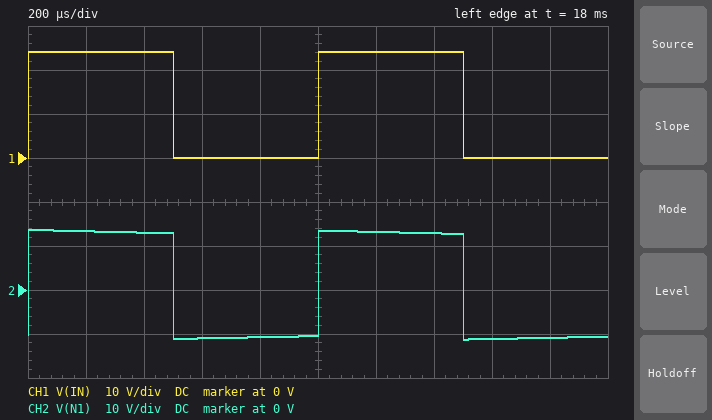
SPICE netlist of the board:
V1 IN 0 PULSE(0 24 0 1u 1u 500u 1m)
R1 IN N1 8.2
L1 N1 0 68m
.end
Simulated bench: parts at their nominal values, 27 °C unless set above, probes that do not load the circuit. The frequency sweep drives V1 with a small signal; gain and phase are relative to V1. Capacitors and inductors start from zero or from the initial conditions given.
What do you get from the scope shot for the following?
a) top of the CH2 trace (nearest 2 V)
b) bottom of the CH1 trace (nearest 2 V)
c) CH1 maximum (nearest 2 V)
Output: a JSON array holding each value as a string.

["14 V", "0 V", "24 V"]
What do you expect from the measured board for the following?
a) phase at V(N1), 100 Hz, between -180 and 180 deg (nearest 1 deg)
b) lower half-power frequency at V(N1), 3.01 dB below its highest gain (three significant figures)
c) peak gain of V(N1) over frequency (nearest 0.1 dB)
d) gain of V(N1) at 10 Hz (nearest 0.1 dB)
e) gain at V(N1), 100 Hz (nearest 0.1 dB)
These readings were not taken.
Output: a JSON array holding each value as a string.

["11 deg", "19.2 Hz", "0 dB", "-6.7 dB", "-0.2 dB"]
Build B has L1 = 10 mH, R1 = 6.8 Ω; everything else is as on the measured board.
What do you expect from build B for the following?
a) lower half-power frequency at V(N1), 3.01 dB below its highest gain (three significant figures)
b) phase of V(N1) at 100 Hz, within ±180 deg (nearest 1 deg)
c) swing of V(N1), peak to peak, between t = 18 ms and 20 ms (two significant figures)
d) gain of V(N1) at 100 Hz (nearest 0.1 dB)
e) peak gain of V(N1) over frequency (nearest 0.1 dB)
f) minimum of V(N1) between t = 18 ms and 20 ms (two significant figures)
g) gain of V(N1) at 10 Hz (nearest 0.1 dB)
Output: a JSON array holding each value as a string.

["108 Hz", "47 deg", "28 V", "-3.4 dB", "0 dB", "-14 V", "-20.7 dB"]
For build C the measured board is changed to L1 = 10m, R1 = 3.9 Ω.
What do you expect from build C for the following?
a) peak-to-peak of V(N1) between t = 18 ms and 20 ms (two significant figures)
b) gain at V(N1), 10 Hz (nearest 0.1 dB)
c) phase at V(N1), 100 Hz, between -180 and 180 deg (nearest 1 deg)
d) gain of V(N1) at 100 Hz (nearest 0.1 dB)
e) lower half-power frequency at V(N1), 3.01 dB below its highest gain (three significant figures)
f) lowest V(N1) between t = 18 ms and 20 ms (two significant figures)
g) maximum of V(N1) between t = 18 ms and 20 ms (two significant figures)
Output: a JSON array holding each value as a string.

["26 V", "-16.0 dB", "32 deg", "-1.4 dB", "62.1 Hz", "-13 V", "13 V"]
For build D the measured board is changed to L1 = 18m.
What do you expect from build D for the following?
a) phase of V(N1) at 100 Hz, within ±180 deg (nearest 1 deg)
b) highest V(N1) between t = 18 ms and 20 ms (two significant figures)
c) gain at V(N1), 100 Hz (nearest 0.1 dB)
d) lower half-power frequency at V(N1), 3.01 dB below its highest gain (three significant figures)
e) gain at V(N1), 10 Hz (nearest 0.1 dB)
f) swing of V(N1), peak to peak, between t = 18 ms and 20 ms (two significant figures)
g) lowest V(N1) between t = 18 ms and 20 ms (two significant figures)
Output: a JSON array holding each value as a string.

["36 deg", "13 V", "-1.8 dB", "72.5 Hz", "-17.3 dB", "27 V", "-13 V"]
